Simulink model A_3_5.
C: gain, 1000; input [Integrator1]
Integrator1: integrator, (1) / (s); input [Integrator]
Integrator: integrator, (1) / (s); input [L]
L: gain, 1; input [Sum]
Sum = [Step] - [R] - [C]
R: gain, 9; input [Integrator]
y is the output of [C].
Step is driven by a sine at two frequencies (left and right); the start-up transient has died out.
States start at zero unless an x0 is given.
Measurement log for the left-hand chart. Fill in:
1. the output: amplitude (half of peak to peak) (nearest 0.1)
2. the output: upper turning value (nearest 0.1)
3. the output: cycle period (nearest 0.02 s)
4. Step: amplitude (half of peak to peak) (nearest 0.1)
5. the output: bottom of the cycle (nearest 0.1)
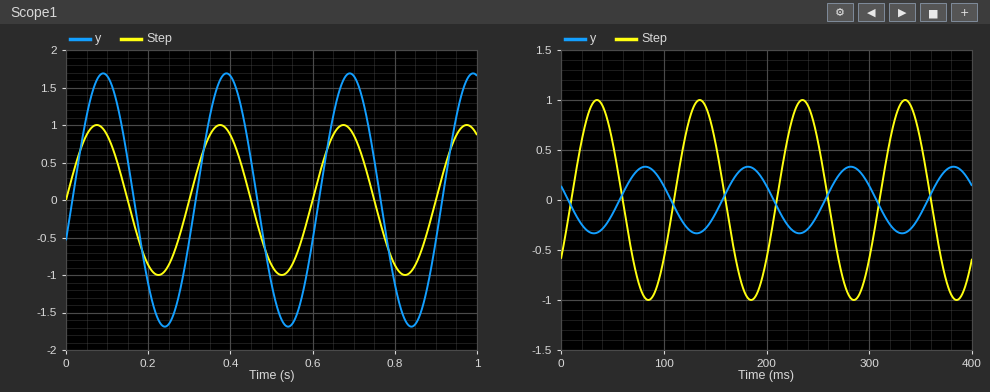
1.7
1.7
0.30 s
1.0
-1.7
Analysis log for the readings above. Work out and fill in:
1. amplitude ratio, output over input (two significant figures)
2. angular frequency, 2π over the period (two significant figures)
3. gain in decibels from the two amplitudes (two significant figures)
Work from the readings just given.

1.7
21 rad/s
4.6 dB
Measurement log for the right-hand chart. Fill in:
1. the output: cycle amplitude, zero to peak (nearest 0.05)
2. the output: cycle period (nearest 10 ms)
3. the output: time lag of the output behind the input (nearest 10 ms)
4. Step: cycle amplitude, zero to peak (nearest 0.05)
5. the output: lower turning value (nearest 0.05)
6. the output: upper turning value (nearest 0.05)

0.35
100 ms
50 ms
1.00
-0.35
0.35
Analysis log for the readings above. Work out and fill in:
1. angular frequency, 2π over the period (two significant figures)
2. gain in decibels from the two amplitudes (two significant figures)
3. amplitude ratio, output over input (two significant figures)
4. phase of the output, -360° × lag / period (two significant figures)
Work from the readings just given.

0.063 rad/ms
-9.1 dB
0.35
-180°
